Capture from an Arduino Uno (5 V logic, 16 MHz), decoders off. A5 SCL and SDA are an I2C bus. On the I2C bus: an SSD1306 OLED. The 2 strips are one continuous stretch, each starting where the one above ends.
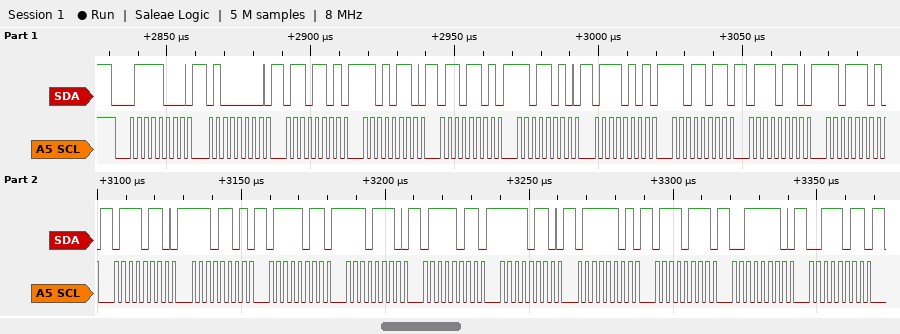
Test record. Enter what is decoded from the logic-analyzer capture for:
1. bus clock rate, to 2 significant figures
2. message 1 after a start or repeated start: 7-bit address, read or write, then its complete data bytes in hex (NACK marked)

400 kHz
0x3C write: 40 6D D6 6D DA 75 DB 76 DD 76 ED 7B EE 7B F6 7D 77 3E 3B
